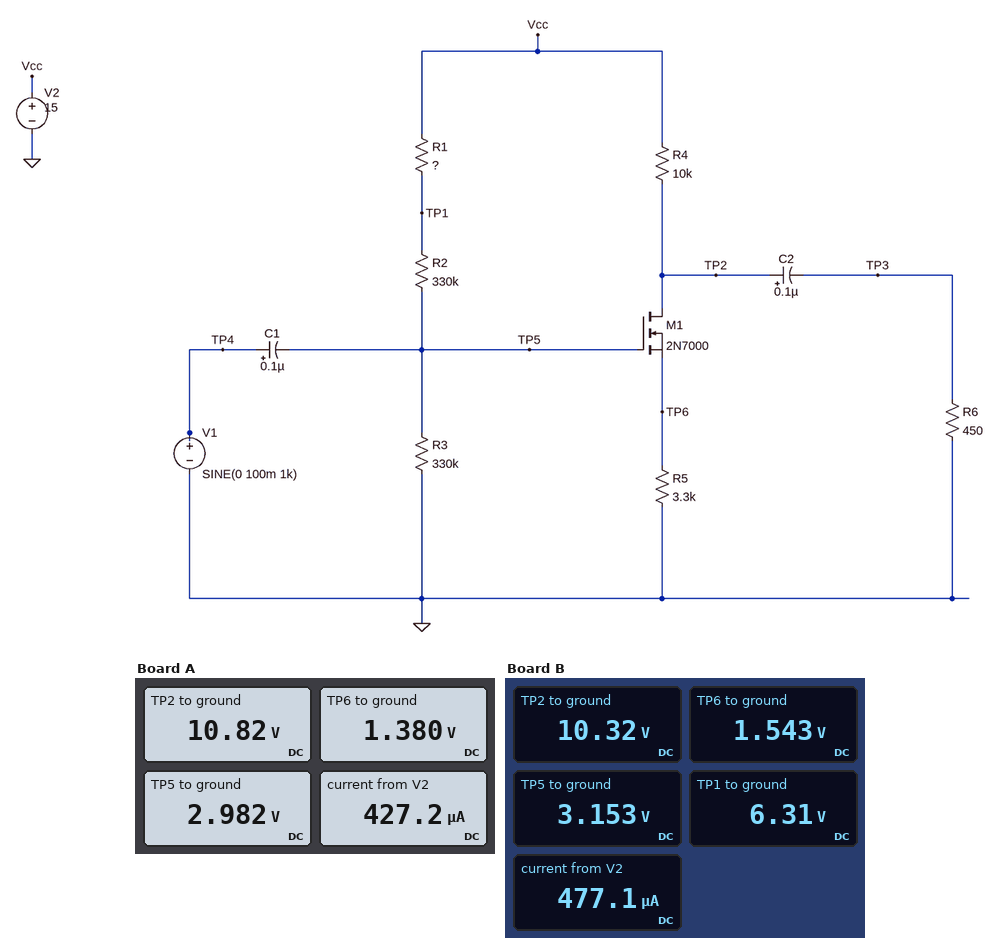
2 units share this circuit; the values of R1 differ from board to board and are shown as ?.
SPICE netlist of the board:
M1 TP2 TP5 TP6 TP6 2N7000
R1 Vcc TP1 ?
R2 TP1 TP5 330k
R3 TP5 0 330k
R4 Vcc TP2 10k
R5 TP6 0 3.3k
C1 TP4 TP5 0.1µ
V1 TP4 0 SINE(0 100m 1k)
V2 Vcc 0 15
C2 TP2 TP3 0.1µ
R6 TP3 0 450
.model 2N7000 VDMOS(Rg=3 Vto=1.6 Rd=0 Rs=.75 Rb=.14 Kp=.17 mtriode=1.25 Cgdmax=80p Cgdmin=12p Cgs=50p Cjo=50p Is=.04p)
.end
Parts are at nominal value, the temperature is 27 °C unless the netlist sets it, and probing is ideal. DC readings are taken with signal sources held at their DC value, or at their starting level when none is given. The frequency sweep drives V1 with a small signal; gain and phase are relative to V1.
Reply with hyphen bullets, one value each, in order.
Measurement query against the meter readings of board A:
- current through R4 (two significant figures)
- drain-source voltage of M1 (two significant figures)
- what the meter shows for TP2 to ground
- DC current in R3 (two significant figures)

- 420 µA
- 9.4 V
- 10.82 V
- 9.0 µA
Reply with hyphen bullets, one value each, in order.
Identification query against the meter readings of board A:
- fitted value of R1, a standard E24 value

- 1 MΩ
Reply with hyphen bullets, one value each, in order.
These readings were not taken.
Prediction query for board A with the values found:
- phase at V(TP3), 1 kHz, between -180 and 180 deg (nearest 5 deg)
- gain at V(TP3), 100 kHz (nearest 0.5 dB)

- -170 deg
- -18.0 dB
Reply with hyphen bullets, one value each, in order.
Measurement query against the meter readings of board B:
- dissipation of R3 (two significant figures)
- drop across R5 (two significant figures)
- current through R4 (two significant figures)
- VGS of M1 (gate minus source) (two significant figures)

- 30 µW
- 1.5 V
- 470 µA
- 1.6 V
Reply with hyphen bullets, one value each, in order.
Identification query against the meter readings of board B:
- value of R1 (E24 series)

- 910 kΩ
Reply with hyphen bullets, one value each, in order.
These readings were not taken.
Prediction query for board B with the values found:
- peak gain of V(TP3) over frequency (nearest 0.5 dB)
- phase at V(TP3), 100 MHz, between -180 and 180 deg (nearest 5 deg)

- 0 dB
- 10 deg
